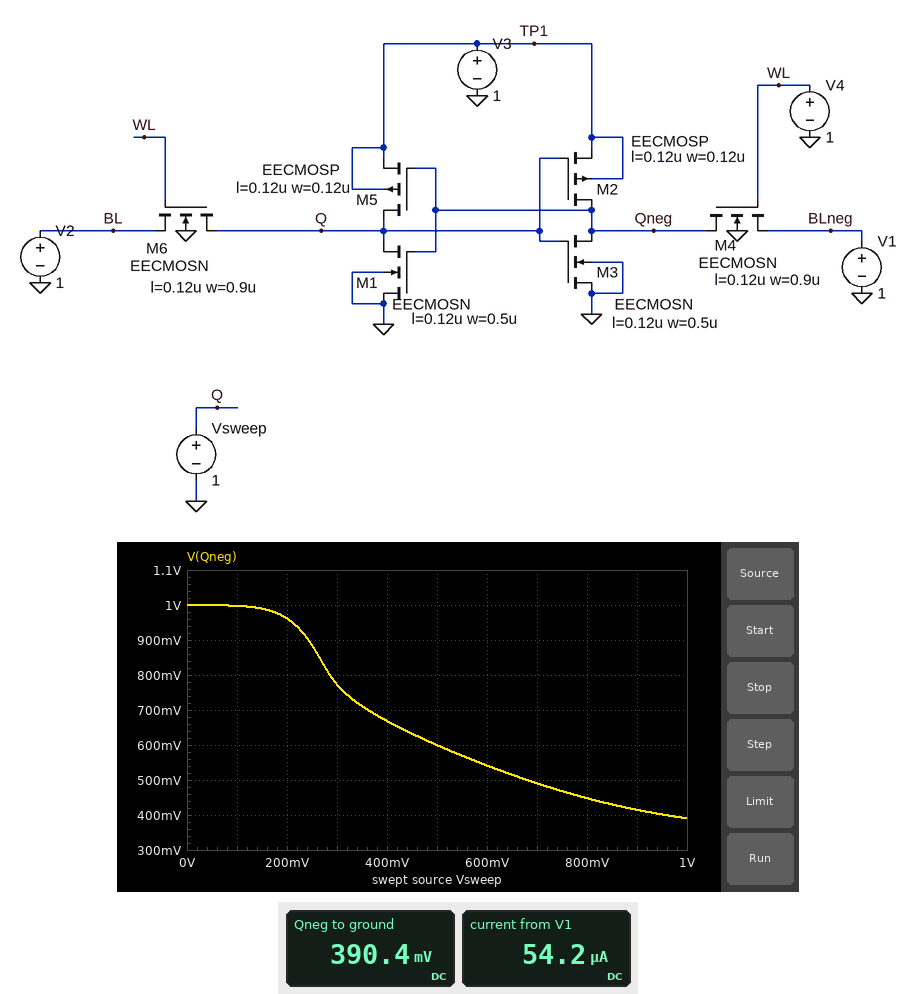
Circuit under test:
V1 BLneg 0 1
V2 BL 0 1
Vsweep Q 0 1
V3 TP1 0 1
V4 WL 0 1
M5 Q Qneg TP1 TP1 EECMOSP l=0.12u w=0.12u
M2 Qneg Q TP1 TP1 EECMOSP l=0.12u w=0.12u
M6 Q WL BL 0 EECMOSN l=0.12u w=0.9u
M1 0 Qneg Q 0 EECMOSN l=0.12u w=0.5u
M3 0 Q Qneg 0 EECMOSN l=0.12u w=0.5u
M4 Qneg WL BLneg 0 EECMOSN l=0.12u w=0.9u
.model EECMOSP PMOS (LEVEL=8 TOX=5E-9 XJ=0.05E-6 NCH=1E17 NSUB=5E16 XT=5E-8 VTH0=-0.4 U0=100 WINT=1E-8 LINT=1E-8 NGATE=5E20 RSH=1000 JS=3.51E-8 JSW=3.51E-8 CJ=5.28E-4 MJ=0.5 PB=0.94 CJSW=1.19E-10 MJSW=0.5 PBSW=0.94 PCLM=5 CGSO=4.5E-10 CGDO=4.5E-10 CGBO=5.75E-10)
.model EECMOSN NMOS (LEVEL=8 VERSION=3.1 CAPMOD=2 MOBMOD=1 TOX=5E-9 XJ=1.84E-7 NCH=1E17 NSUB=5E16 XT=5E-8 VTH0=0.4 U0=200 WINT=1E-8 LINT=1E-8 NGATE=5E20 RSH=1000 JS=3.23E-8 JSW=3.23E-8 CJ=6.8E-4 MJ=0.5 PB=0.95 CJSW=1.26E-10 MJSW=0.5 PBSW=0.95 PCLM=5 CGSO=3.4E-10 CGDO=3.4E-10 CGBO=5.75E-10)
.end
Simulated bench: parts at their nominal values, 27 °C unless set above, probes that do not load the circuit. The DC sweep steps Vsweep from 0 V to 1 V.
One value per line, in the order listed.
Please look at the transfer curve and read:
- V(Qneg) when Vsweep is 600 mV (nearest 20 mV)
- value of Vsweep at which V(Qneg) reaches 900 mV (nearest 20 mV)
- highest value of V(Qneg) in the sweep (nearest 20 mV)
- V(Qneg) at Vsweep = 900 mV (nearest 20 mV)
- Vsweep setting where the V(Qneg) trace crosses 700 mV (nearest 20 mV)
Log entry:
540 mV
240 mV
1.00 V
420 mV
360 mV
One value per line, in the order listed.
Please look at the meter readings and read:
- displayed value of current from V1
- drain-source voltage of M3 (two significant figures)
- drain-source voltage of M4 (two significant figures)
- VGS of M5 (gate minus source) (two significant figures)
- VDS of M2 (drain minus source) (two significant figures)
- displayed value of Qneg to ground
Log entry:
54.2 µA
-390 mV
-610 mV
-610 mV
-610 mV
390.4 mV
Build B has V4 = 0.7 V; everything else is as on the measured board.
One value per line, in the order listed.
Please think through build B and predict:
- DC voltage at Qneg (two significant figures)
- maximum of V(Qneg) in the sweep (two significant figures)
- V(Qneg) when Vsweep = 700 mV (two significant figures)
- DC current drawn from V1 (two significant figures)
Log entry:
230 mV
1.0 V
280 mV
36 µA
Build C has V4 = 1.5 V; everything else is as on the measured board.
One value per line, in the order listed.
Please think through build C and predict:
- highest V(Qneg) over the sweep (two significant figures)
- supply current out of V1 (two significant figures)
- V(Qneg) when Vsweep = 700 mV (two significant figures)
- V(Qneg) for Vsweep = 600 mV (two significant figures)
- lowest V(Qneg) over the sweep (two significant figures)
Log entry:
1.0 V
70 µA
760 mV
810 mV
640 mV
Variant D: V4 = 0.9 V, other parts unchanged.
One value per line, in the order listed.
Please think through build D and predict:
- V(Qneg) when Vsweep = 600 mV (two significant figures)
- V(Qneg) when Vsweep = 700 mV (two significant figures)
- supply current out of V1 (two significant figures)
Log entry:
470 mV
420 mV
49 µA
